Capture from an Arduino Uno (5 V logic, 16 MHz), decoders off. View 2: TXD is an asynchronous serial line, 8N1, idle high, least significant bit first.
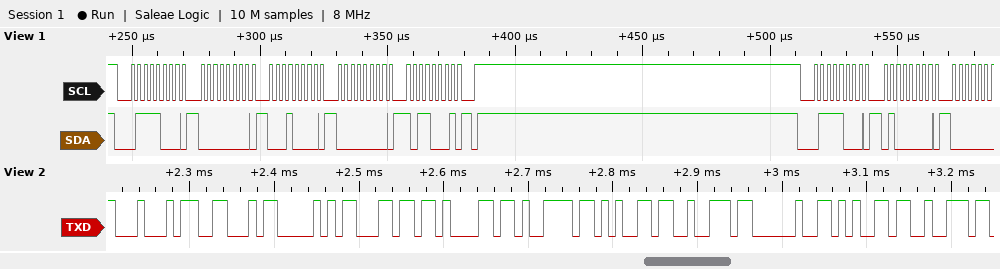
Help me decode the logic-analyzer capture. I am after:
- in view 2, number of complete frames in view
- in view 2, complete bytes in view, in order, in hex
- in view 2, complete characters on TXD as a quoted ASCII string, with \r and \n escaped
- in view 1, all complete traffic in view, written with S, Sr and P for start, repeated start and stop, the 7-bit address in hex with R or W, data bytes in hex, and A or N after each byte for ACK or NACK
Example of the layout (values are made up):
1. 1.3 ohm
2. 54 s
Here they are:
1. 11
2. 44 46 50 6C 61 79 65 72 20 65 72
3. "DFPlayer er"
4. S 3CW A 00 A 10 A 00 A B1 A P S 3CW A 40 A
